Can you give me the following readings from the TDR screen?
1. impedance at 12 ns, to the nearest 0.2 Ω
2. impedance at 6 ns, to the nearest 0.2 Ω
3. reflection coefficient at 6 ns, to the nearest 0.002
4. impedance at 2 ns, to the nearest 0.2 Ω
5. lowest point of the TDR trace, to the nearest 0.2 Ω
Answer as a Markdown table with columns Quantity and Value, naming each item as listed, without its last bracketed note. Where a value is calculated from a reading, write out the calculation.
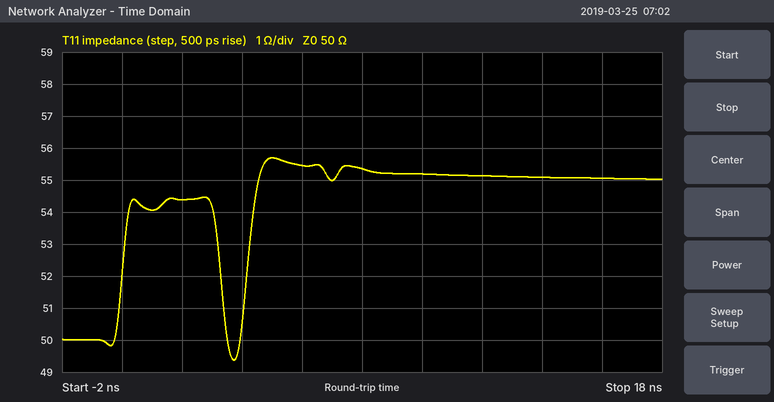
| Quantity | Value |
|---|---|
| impedance at 12 ns, to the nearest 0.2 Ω | 55.2 Ω |
| impedance at 6 ns, to the nearest 0.2 Ω | 55.4 Ω |
| reflection coefficient at 6 ns, to the nearest 0.002 | (55.4 − 50)/(55.4 + 50) ≈ +0.0512, so +0.052 to the nearest 0.002 |
| impedance at 2 ns, to the nearest 0.2 Ω | 54.4 Ω |
| lowest point of the TDR trace, to the nearest 0.2 Ω | 49.4 Ω |
